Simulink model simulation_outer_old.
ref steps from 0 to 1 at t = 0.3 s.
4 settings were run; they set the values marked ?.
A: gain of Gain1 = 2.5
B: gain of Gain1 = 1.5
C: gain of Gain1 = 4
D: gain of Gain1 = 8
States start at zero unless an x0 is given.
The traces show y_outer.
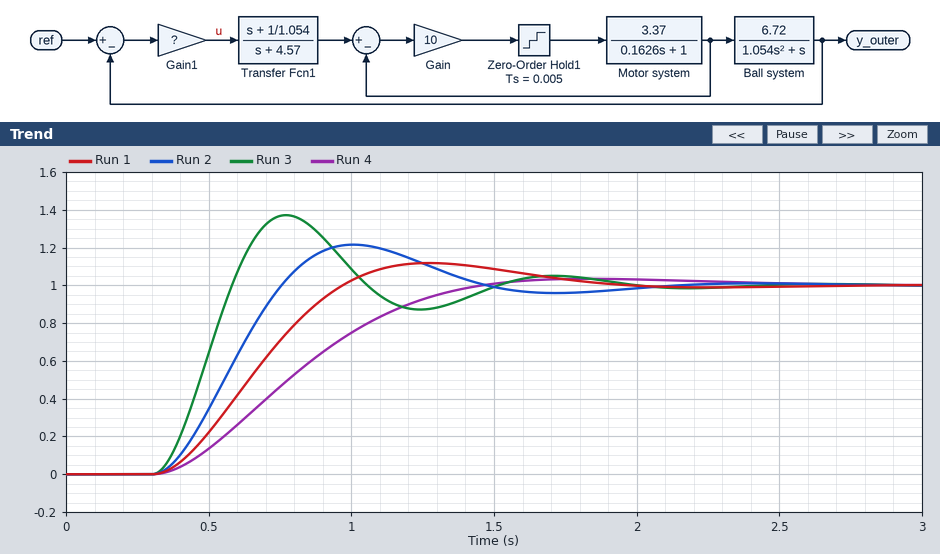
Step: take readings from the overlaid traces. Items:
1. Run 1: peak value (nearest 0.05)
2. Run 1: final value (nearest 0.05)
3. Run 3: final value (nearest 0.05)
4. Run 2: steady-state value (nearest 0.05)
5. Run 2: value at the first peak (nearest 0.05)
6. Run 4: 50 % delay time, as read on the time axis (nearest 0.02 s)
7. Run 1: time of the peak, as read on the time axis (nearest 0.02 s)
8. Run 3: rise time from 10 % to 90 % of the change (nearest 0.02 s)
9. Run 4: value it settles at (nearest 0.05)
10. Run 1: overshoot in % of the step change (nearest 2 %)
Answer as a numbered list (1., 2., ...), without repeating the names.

1. 1.10
2. 1.00
3. 1.00
4. 1.00
5. 1.20
6. 0.78 s
7. 1.28 s
8. 0.18 s
9. 1.00
10. 12 %
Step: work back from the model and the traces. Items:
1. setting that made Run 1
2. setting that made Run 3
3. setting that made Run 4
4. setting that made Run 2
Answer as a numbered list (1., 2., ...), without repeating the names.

1. A
2. D
3. B
4. C
